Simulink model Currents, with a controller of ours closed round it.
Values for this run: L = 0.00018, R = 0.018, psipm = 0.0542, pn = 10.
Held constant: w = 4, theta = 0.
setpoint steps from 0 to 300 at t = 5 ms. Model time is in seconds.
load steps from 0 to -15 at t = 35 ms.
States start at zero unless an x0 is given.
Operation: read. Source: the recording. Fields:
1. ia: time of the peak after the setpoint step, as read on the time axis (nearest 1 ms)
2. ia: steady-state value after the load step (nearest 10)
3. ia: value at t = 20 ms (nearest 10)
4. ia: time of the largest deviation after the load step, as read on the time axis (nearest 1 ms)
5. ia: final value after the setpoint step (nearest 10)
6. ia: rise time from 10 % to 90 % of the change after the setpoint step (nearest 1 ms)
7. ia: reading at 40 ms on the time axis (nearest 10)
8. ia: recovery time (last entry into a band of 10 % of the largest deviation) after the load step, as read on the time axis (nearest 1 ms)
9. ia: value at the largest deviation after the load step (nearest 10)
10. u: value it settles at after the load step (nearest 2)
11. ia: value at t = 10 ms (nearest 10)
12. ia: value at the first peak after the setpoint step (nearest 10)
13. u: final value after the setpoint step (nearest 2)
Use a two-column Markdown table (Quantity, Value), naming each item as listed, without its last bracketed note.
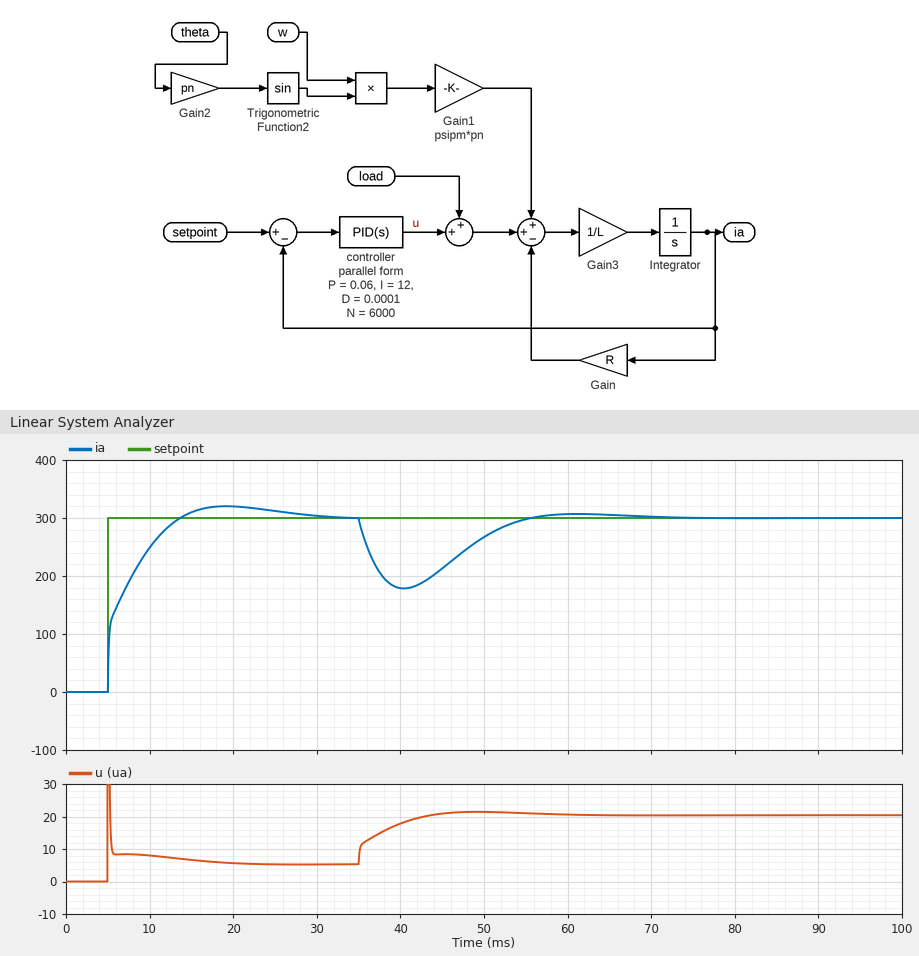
| Quantity | Value |
|---|---|
| ia: time of the peak after the setpoint step, as read on the time axis | 19 ms |
| ia: steady-state value after the load step | 300 |
| ia: value at t = 20 ms | 320 |
| ia: time of the largest deviation after the load step, as read on the time axis | 40 ms |
| ia: final value after the setpoint step | 300 |
| ia: rise time from 10 % to 90 % of the change after the setpoint step | 6 ms |
| ia: reading at 40 ms on the time axis | 180 |
| ia: recovery time (last entry into a band of 10 % of the largest deviation) after the load step, as read on the time axis | 53 ms |
| ia: value at the largest deviation after the load step | 180 |
| u: value it settles at after the load step | 20 |
| ia: value at t = 10 ms | 250 |
| ia: value at the first peak after the setpoint step | 320 |
| u: final value after the setpoint step | 6 |
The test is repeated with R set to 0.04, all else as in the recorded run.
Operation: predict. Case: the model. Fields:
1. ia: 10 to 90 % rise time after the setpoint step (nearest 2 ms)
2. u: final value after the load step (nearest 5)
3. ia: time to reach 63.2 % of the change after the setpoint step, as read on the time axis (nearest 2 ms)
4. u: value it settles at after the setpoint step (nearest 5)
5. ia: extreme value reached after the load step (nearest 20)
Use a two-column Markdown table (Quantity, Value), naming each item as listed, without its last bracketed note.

| Quantity | Value |
|---|---|
| ia: 10 to 90 % rise time after the setpoint step | 10 ms |
| u: final value after the load step | 25 |
| ia: time to reach 63.2 % of the change after the setpoint step, as read on the time axis | 8 ms |
| u: value it settles at after the setpoint step | 10 |
| ia: extreme value reached after the load step | 200 |
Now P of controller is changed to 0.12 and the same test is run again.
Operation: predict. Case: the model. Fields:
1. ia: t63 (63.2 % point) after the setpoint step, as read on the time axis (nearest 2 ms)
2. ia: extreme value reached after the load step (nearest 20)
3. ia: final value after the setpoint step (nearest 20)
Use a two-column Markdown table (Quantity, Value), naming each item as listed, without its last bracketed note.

| Quantity | Value |
|---|---|
| ia: t63 (63.2 % point) after the setpoint step, as read on the time axis | 6 ms |
| ia: extreme value reached after the load step | 220 |
| ia: final value after the setpoint step | 300 |
